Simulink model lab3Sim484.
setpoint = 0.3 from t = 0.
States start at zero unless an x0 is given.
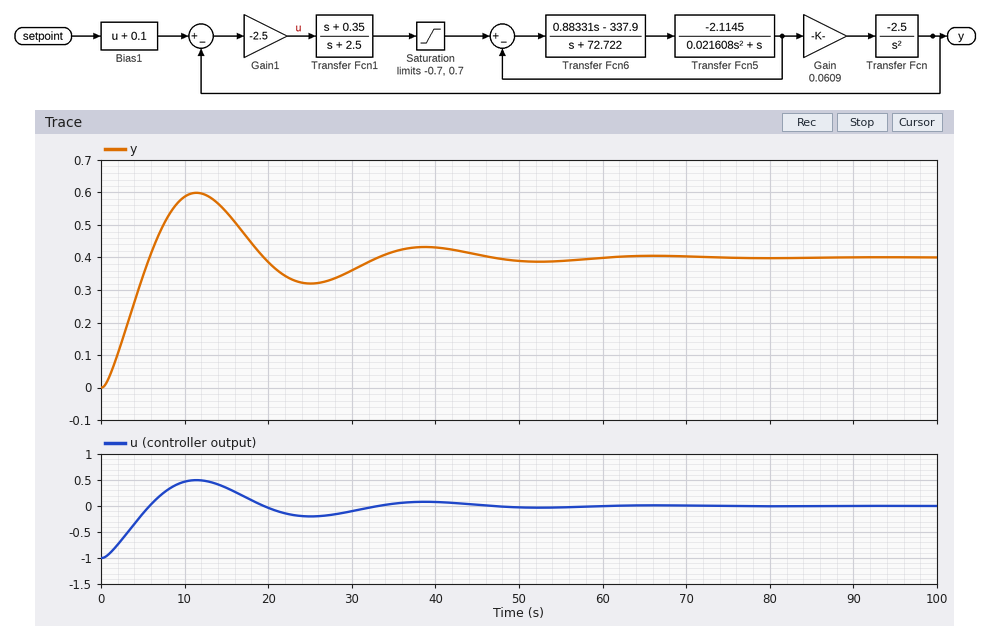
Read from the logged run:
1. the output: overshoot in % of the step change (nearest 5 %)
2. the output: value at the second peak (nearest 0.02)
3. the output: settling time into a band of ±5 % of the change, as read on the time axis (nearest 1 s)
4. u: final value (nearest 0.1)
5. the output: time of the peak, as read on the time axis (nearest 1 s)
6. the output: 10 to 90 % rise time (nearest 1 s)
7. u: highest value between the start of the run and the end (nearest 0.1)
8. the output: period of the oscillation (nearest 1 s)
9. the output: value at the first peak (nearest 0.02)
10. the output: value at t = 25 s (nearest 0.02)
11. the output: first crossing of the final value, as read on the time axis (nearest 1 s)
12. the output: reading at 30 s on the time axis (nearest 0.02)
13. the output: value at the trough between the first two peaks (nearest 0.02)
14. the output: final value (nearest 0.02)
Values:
50 %
0.44
43 s
0.0
11 s
4 s
0.5
27 s
0.60
0.32
6 s
0.36
0.32
0.40
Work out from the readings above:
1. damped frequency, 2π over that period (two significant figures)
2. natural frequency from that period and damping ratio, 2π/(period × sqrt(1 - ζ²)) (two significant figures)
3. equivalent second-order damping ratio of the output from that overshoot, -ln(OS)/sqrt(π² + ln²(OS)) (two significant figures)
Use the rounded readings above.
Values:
0.23 rad/s
0.24 rad/s
0.22
